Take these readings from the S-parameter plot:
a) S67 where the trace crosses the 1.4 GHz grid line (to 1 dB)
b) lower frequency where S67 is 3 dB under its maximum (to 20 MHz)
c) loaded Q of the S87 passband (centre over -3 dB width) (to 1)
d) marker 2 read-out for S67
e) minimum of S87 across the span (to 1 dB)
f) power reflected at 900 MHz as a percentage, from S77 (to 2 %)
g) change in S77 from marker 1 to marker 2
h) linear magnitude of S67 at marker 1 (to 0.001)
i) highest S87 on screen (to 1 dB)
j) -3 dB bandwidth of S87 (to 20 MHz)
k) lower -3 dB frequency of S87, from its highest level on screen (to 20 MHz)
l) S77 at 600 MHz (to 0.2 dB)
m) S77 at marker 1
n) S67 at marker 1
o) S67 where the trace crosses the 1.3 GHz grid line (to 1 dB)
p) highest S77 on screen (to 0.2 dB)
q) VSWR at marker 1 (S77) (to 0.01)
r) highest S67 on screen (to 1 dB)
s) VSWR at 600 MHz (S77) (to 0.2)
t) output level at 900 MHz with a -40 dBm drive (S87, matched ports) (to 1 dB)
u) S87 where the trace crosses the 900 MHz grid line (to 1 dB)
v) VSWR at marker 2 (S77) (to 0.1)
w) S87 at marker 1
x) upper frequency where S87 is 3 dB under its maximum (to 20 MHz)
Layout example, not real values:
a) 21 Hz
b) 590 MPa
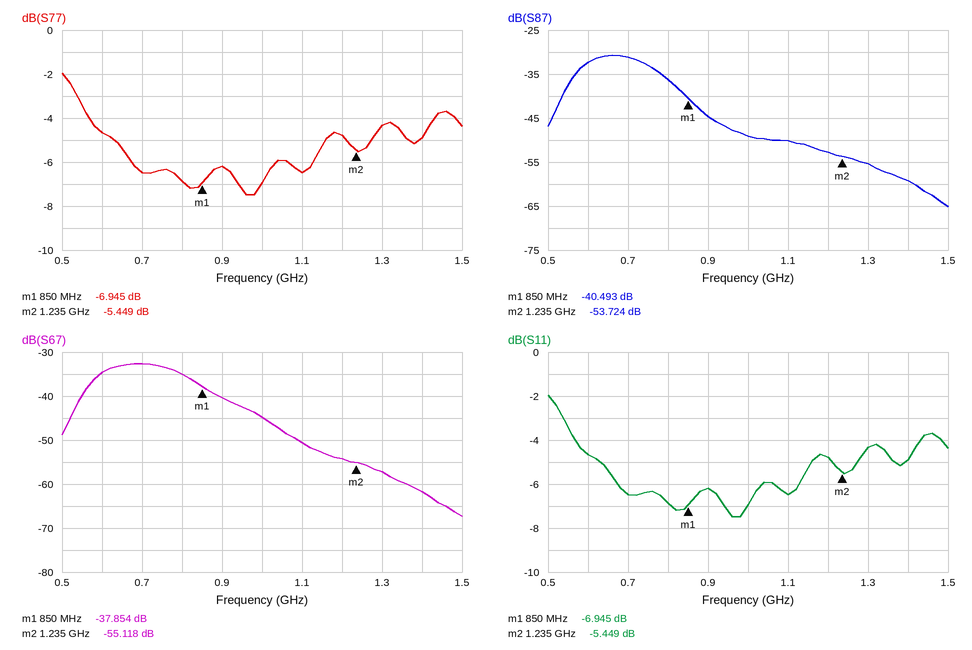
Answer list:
a) -62 dB
b) 580 MHz
c) 4
d) -55.118 dB
e) -65 dB
f) 24 %
g) 1.496 dB
h) 0.013
i) -31 dB
j) 180 MHz
k) 580 MHz
l) -4.6 dB
m) -6.945 dB
n) -37.854 dB
o) -57 dB
p) -2.0 dB
q) 2.63
r) -33 dB
s) 3.8
t) -85 dBm
u) -45 dB
v) 3.3
w) -40.493 dB
x) 760 MHz
